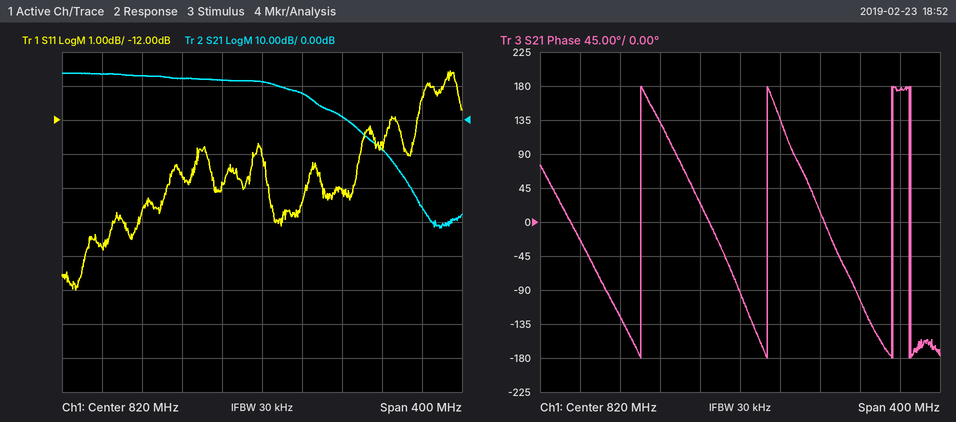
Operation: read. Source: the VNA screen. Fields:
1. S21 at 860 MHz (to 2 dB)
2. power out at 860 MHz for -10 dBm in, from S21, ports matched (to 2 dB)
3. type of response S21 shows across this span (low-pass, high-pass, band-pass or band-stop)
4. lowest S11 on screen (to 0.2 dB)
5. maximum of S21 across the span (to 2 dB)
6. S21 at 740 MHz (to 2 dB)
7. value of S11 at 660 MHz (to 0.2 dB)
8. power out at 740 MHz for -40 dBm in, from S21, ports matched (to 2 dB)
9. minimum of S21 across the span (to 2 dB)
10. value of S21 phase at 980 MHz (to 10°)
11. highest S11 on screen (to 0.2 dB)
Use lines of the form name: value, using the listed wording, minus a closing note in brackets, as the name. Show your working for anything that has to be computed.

S21 at 860 MHz: 8 dB
power out at 860 MHz for -10 dBm in, from S21, ports matched: -10 dBm + (8 dB) = -2 dBm
type of response S21 shows across this span: low-pass
lowest S11 on screen: -17.0 dB
maximum of S21 across the span: 14 dB
S21 at 740 MHz: 12 dB
value of S11 at 660 MHz: -15.8 dB
power out at 740 MHz for -40 dBm in, from S21, ports matched: -40 dBm + (12 dB) = -28 dBm
minimum of S21 across the span: -32 dB
value of S21 phase at 980 MHz: 180°
highest S11 on screen: -10.6 dB
